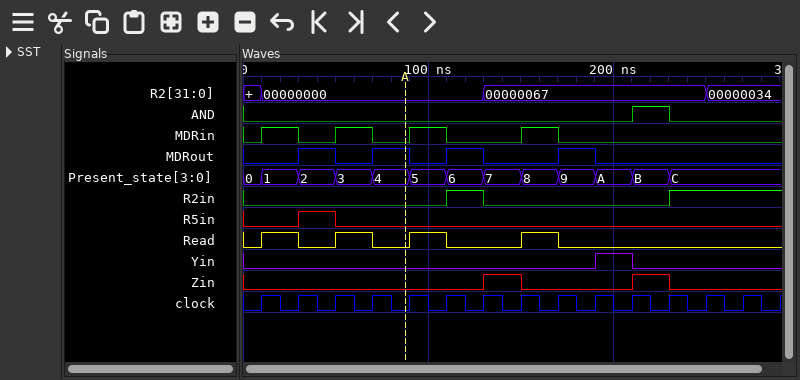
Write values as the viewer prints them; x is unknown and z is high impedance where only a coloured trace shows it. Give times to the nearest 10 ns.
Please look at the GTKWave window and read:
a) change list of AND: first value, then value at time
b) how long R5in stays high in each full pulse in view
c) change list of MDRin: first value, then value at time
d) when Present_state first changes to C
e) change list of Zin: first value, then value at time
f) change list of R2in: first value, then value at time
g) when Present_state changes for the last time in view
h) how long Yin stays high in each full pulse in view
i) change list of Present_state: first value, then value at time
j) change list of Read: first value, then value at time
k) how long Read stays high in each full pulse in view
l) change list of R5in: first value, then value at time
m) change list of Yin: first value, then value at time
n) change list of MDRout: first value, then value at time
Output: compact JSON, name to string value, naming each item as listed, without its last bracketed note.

{"change list of AND: first value, then value at time": "0, 1 at 210 ns, 0 at 230 ns", "how long R5in stays high in each full pulse in view": "20 ns", "change list of MDRin: first value, then value at time": "0, 1 at 10 ns, 0 at 30 ns, 1 at 50 ns, 0 at 70 ns, 1 at 90 ns, 0 at 110 ns, 1 at 150 ns, 0 at 170 ns", "when Present_state first changes to C": "230 ns", "change list of Zin: first value, then value at time": "0, 1 at 130 ns, 0 at 150 ns, 1 at 210 ns, 0 at 230 ns", "change list of R2in: first value, then value at time": "0, 1 at 110 ns, 0 at 130 ns, 1 at 230 ns", "when Present_state changes for the last time in view": "230 ns", "how long Yin stays high in each full pulse in view": "20 ns", "change list of Present_state: first value, then value at time": "0, 1 at 10 ns, 2 at 30 ns, 3 at 50 ns, 4 at 70 ns, 5 at 90 ns, 6 at 110 ns, 7 at 130 ns, 8 at 150 ns, 9 at 170 ns, A at 190 ns, B at 210 ns, C at 230 ns", "change list of Read: first value, then value at time": "0, 1 at 10 ns, 0 at 30 ns, 1 at 50 ns, 0 at 70 ns, 1 at 90 ns, 0 at 110 ns, 1 at 150 ns, 0 at 170 ns", "how long Read stays high in each full pulse in view": "20 ns, 20 ns, 20 ns, 20 ns", "change list of R5in: first value, then value at time": "0, 1 at 30 ns, 0 at 50 ns", "change list of Yin: first value, then value at time": "0, 1 at 190 ns, 0 at 210 ns", "change list of MDRout: first value, then value at time": "0, 1 at 30 ns, 0 at 50 ns, 1 at 70 ns, 0 at 90 ns, 1 at 110 ns, 0 at 130 ns, 1 at 170 ns, 0 at 190 ns"}
